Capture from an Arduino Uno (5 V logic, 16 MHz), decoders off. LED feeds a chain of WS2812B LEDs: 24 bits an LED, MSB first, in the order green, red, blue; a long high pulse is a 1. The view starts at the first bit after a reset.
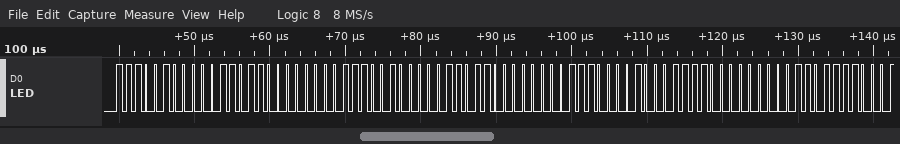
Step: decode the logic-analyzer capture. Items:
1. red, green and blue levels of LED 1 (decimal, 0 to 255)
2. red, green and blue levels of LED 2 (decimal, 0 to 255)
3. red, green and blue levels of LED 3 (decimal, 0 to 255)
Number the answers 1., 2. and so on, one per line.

1. 27, 228, 0
2. 27, 228, 0
3. 30, 225, 0
